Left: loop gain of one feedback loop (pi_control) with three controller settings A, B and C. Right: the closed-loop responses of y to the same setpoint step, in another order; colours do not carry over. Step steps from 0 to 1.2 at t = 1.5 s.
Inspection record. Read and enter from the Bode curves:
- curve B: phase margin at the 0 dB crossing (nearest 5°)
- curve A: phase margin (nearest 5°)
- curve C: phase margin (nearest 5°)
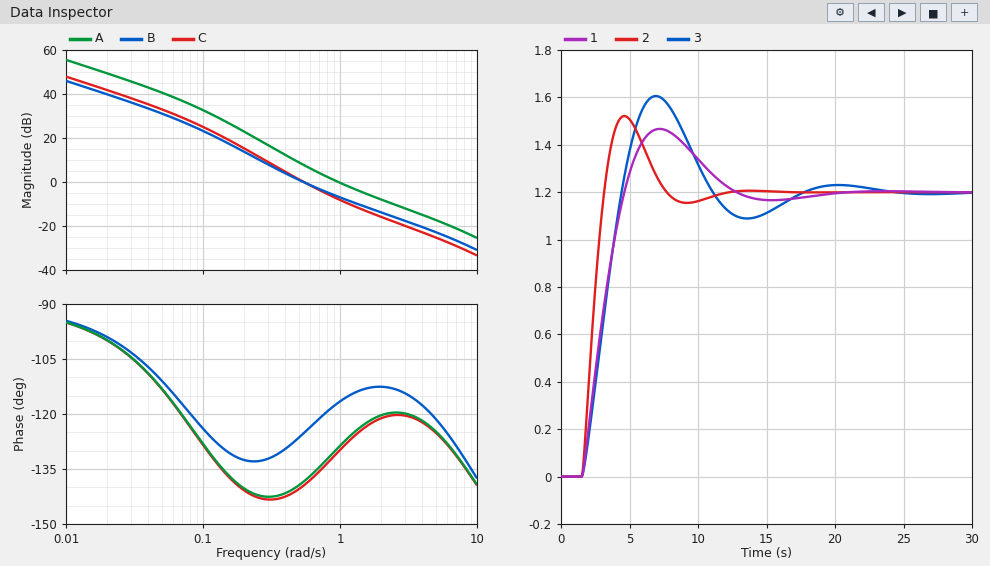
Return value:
55°
50°
40°
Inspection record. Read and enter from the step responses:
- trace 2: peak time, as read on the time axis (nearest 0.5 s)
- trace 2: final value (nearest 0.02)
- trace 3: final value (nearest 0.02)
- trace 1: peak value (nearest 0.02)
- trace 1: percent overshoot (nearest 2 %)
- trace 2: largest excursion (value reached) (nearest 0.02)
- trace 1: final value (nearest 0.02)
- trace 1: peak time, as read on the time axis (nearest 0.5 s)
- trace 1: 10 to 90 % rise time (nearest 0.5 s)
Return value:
4.5 s
1.20
1.20
1.46
22 %
1.52
1.20
7.0 s
2.5 s
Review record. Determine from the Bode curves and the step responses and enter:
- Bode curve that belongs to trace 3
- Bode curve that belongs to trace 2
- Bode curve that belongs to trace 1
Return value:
C
A
B
